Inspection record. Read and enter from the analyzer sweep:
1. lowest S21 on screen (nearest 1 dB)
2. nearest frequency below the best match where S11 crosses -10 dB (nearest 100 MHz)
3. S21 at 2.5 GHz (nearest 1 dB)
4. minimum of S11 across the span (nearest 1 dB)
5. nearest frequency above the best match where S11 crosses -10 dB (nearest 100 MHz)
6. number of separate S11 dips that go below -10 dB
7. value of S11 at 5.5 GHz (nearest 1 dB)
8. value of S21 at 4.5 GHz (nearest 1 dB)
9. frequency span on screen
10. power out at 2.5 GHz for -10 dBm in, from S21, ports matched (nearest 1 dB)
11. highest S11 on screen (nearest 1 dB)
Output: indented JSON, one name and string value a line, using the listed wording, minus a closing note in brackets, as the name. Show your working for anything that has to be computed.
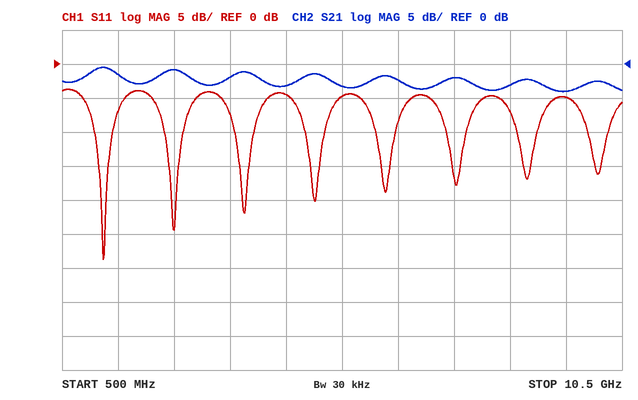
{
  "lowest S21 on screen": "-4 dB",
  "nearest frequency below the best match where S11 crosses -10 dB": "1.1 GHz",
  "S21 at 2.5 GHz": "-1 dB",
  "minimum of S11 across the span": "-29 dB",
  "nearest frequency above the best match where S11 crosses -10 dB": "1.4 GHz",
  "number of separate S11 dips that go below -10 dB": "8",
  "value of S11 at 5.5 GHz": "-5 dB",
  "value of S21 at 4.5 GHz": "-3 dB",
  "frequency span on screen": "10 GHz",
  "power out at 2.5 GHz for -10 dBm in, from S21, ports matched": "-10 dBm + (-1 dB) = -11 dBm",
  "highest S11 on screen": "-4 dB"
}
